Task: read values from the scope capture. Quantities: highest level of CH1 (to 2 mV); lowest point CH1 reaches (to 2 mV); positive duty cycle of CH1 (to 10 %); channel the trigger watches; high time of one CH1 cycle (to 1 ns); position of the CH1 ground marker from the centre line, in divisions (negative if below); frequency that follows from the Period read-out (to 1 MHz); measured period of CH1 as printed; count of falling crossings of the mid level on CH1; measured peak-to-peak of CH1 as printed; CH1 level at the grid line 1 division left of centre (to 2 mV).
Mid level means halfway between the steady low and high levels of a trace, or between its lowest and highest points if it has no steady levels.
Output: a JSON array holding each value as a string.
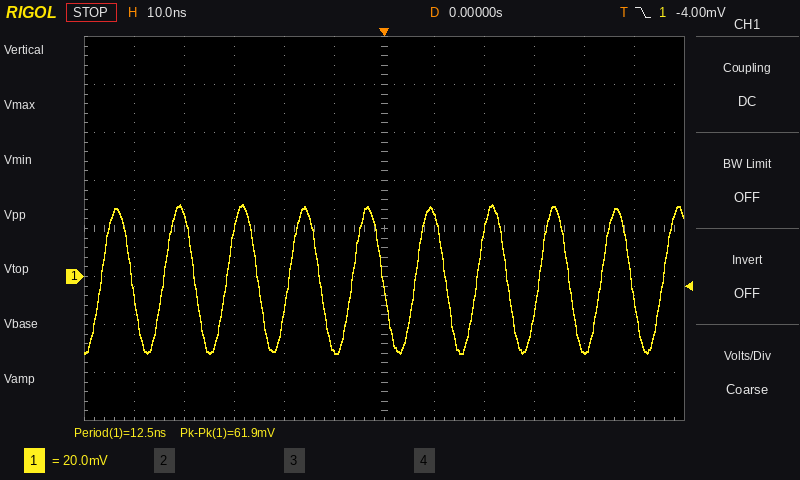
["30 mV", "-32 mV", "50 %", "CH1", "6 ns", "-1.0 div", "80 MHz", "12.5 ns", "9", "61.9 mV", "-30 mV"]
